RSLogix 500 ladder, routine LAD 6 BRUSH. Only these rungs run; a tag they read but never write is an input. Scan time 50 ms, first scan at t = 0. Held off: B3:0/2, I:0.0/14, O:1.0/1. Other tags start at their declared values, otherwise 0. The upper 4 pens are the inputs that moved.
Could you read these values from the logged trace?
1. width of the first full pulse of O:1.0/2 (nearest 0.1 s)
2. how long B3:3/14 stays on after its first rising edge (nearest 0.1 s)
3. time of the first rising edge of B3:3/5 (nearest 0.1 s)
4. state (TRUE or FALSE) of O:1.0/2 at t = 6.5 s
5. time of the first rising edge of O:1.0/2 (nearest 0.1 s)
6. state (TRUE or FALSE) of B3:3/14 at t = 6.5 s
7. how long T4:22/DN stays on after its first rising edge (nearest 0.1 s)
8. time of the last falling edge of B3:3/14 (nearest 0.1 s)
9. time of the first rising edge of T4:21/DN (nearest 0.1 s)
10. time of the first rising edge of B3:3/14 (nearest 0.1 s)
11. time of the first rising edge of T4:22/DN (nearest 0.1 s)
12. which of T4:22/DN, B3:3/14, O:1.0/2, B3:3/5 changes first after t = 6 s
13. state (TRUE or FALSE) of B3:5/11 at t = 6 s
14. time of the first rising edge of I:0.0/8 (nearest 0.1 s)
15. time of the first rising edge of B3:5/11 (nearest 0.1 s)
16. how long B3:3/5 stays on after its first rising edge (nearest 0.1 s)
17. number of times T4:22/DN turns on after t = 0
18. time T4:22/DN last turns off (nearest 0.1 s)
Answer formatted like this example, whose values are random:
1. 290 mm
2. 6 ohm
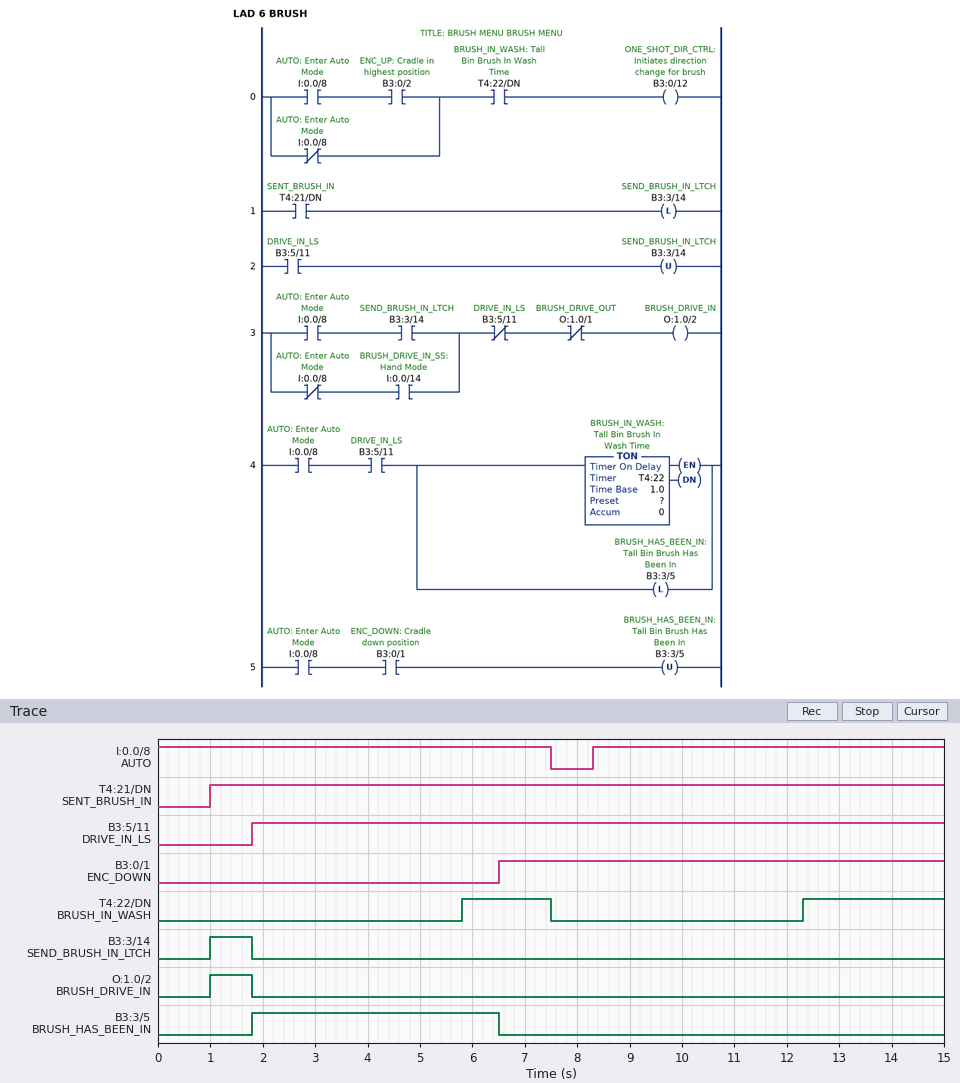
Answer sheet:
1. 0.8 s
2. 0.8 s
3. 1.8 s
4. FALSE
5. 1.0 s
6. FALSE
7. 1.7 s
8. 1.8 s
9. 1.0 s
10. 1.0 s
11. 5.8 s
12. B3:3/5
13. TRUE
14. 8.3 s
15. 1.8 s
16. 4.7 s
17. 2
18. 7.5 s
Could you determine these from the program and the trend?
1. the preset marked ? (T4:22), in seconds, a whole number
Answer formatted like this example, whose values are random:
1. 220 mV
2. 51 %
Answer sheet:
1. 4 s
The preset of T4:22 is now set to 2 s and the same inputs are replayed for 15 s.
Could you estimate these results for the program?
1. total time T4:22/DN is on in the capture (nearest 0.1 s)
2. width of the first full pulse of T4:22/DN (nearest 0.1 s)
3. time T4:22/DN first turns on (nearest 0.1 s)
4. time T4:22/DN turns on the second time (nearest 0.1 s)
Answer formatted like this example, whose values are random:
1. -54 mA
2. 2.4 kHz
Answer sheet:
1. 8.4 s
2. 3.7 s
3. 3.8 s
4. 10.3 s
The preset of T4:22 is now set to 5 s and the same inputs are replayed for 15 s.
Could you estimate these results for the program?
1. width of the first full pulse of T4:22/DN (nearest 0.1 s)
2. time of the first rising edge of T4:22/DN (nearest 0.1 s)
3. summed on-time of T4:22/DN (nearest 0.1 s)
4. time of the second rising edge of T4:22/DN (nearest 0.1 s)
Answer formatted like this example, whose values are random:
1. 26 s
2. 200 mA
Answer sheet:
1. 0.7 s
2. 6.8 s
3. 2.4 s
4. 13.3 s
